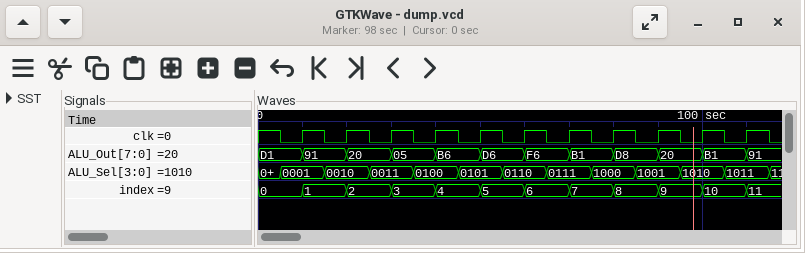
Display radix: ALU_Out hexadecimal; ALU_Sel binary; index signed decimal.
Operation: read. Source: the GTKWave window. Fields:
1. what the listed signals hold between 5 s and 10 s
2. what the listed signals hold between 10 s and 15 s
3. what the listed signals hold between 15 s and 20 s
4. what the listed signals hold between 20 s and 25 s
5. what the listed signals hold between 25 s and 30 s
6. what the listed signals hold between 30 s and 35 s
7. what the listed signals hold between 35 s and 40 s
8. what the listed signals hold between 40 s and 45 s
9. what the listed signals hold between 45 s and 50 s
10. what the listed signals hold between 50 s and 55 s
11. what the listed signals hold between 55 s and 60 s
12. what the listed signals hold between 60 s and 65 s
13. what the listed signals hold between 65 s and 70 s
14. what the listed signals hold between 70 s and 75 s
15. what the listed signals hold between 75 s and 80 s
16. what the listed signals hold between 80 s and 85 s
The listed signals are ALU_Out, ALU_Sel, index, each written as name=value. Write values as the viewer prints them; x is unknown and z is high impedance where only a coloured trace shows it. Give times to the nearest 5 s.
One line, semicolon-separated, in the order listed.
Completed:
ALU_Out=D1, ALU_Sel=0001, index=0; ALU_Out=91, ALU_Sel=0001, index=1; ALU_Out=91, ALU_Sel=0010, index=1; ALU_Out=20, ALU_Sel=0010, index=2; ALU_Out=20, ALU_Sel=0011, index=2; ALU_Out=05, ALU_Sel=0011, index=3; ALU_Out=05, ALU_Sel=0100, index=3; ALU_Out=B6, ALU_Sel=0100, index=4; ALU_Out=B6, ALU_Sel=0101, index=4; ALU_Out=D6, ALU_Sel=0101, index=5; ALU_Out=D6, ALU_Sel=0110, index=5; ALU_Out=F6, ALU_Sel=0110, index=6; ALU_Out=F6, ALU_Sel=0111, index=6; ALU_Out=B1, ALU_Sel=0111, index=7; ALU_Out=B1, ALU_Sel=1000, index=7; ALU_Out=D8, ALU_Sel=1000, index=8
